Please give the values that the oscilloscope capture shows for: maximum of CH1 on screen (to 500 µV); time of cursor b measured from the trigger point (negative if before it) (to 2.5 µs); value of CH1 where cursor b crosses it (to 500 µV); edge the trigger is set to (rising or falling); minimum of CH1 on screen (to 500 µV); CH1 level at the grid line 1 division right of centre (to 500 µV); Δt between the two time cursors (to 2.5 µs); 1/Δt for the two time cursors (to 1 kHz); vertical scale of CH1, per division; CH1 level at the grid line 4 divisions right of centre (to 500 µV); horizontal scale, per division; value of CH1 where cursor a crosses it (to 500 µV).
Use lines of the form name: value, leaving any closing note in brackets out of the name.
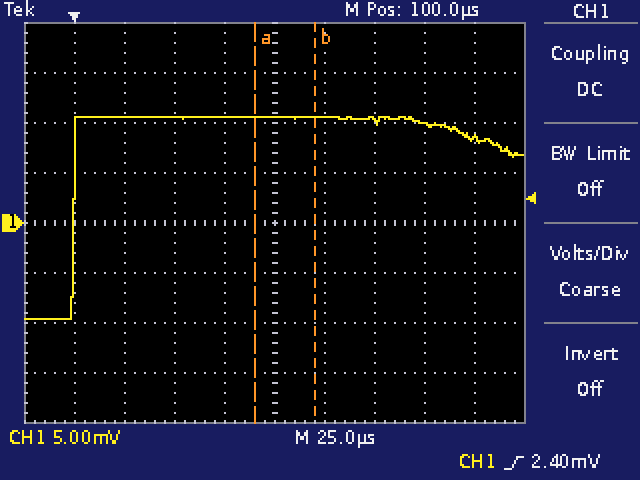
maximum of CH1 on screen: 10.5 mV
time of cursor b measured from the trigger point (negative if before it): +120.0 µs
value of CH1 where cursor b crosses it: 10.5 mV
edge the trigger is set to: rising
minimum of CH1 on screen: -9.5 mV
CH1 level at the grid line 1 division right of centre: 10.5 mV
Δt between the two time cursors: 30.0 µs
1/Δt for the two time cursors: 33 kHz
vertical scale of CH1, per division: 5 mV
CH1 level at the grid line 4 divisions right of centre: 8.5 mV
horizontal scale, per division: 25 µs
value of CH1 where cursor a crosses it: 10.5 mV
